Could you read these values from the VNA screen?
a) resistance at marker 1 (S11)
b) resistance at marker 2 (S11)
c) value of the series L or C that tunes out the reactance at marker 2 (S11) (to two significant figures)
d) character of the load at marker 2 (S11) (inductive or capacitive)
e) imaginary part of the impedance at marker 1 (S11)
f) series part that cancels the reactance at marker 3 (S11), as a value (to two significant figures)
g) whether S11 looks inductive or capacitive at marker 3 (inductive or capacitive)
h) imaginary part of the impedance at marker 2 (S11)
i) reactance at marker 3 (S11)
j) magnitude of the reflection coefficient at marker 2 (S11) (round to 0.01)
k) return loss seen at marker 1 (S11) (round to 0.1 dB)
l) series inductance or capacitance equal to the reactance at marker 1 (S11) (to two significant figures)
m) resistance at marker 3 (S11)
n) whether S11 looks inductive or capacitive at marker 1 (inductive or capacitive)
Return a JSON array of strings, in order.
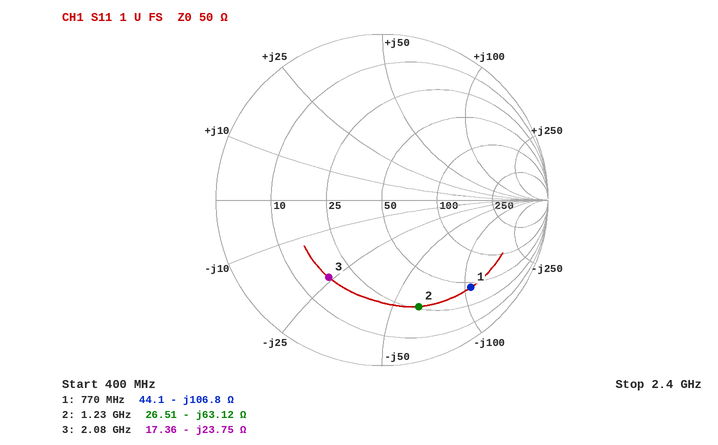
["44.1 Ω", "26.51 Ω", "8.2 nH", "capacitive", "-106.8 Ω", "1.8 nH", "capacitive", "-63.12 Ω", "-23.75 Ω", "0.68", "2.5 dB", "1.9 pF", "17.36 Ω", "capacitive"]
